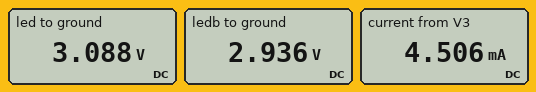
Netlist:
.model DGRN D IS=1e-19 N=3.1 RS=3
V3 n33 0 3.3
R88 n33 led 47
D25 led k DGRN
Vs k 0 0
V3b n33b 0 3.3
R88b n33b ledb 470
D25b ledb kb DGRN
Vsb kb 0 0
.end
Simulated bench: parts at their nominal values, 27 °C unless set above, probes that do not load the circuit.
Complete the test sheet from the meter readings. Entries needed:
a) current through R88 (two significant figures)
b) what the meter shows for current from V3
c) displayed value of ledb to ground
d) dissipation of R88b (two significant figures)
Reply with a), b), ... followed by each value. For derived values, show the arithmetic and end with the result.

a) (3.3 V - 3.088 V) / 47 Ω = 4.5 mA
b) 4.506 mA
c) 2.936 V
d) (3.3 V - 2.936 V)^2 / 470 Ω = 280 µW
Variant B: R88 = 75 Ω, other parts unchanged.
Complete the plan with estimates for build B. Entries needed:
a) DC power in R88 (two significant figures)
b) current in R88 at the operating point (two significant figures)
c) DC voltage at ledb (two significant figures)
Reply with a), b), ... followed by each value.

a) 780 µW
b) 3.2 mA
c) 2.9 V
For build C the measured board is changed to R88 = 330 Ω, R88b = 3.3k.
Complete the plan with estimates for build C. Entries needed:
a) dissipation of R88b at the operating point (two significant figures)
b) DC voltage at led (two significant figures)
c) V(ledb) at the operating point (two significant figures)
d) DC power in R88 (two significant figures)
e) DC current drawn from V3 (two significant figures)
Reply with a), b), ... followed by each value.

a) 75 µW
b) 3.0 V
c) 2.8 V
d) 350 µW
e) 1.0 mA
